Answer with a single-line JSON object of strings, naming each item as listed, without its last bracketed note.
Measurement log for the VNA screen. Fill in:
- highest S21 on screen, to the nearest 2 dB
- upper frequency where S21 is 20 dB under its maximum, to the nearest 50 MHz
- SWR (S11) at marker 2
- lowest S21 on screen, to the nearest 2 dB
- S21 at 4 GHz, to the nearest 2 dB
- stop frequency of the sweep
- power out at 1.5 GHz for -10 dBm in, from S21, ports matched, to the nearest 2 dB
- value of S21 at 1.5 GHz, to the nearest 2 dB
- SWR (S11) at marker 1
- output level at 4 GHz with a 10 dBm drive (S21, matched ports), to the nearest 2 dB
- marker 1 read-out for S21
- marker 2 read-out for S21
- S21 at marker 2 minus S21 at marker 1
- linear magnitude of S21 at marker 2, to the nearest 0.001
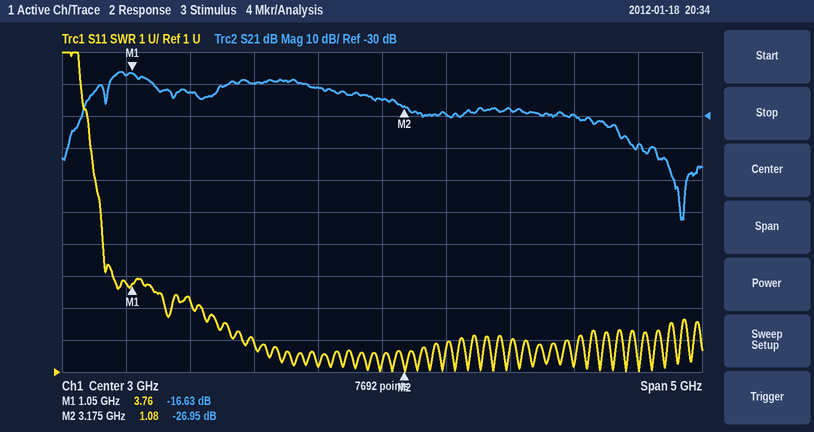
{"highest S21 on screen, to the nearest 2 dB": "-16 dB", "upper frequency where S21 is 20 dB under its maximum, to the nearest 50 MHz": "4.85 GHz", "SWR (S11) at marker 2": "1.08", "lowest S21 on screen, to the nearest 2 dB": "-62 dB", "S21 at 4 GHz, to the nearest 2 dB": "-28 dB", "stop frequency of the sweep": "5.5 GHz", "power out at 1.5 GHz for -10 dBm in, from S21, ports matched, to the nearest 2 dB": "-32 dBm", "value of S21 at 1.5 GHz, to the nearest 2 dB": "-22 dB", "SWR (S11) at marker 1": "3.76", "output level at 4 GHz with a 10 dBm drive (S21, matched ports), to the nearest 2 dB": "-18 dBm", "marker 1 read-out for S21": "-16.63 dB", "marker 2 read-out for S21": "-26.95 dB", "S21 at marker 2 minus S21 at marker 1": "-10.32 dB", "linear magnitude of S21 at marker 2, to the nearest 0.001": "0.045"}
